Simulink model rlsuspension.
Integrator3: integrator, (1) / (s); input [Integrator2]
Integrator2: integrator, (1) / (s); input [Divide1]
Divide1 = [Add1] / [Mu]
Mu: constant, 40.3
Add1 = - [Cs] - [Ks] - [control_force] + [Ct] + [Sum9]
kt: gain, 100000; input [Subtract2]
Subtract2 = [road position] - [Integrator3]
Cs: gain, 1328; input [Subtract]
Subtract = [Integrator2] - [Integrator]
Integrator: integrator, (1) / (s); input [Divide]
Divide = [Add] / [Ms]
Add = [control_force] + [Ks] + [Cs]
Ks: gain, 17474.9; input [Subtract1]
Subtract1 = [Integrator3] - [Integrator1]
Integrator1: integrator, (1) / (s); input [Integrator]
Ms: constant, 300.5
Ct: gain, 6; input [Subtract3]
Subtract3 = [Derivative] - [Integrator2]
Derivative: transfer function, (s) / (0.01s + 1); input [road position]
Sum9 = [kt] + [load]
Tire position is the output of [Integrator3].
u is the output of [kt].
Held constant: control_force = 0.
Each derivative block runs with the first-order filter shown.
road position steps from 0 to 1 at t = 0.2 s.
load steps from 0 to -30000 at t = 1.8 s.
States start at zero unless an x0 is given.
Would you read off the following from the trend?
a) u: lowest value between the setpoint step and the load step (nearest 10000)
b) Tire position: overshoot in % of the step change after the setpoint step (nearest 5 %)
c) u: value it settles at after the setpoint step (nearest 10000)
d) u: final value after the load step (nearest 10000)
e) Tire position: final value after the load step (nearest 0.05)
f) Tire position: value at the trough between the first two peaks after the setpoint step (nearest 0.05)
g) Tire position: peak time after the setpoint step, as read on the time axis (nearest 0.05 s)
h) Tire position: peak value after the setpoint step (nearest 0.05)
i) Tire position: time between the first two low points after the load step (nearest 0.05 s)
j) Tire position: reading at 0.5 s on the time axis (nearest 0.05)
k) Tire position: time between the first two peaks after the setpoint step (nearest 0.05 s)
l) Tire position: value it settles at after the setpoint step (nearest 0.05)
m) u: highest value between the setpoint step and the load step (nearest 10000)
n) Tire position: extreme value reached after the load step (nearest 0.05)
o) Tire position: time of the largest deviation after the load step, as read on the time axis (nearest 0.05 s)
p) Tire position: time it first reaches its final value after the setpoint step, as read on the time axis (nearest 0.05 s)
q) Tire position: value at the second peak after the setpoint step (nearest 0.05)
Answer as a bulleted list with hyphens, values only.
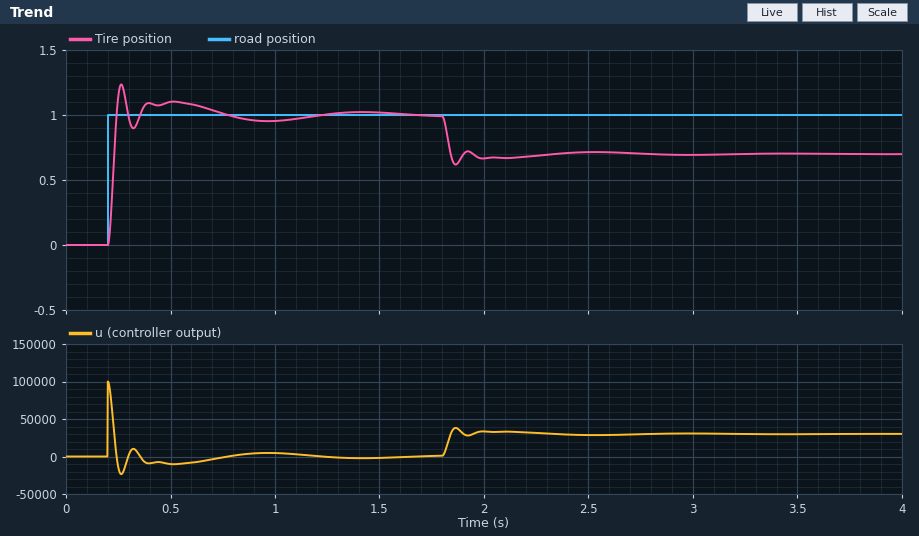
- -20000
- 25 %
- 0
- 30000
- 0.70
- 0.90
- 0.25 s
- 1.25
- 0.15 s
- 1.10
- 0.25 s
- 1.00
- 100000
- 0.60
- 1.85 s
- 0.25 s
- 1.10
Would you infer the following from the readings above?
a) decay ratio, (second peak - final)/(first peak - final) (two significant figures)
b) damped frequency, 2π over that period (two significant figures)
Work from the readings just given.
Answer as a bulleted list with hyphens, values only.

- 0.40
- 25 rad/s
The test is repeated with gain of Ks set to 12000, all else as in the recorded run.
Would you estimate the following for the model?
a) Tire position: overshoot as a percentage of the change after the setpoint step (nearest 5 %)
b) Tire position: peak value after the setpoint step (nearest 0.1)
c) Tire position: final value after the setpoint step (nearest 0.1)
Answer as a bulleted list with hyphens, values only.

- 30 %
- 1.3
- 1.0
